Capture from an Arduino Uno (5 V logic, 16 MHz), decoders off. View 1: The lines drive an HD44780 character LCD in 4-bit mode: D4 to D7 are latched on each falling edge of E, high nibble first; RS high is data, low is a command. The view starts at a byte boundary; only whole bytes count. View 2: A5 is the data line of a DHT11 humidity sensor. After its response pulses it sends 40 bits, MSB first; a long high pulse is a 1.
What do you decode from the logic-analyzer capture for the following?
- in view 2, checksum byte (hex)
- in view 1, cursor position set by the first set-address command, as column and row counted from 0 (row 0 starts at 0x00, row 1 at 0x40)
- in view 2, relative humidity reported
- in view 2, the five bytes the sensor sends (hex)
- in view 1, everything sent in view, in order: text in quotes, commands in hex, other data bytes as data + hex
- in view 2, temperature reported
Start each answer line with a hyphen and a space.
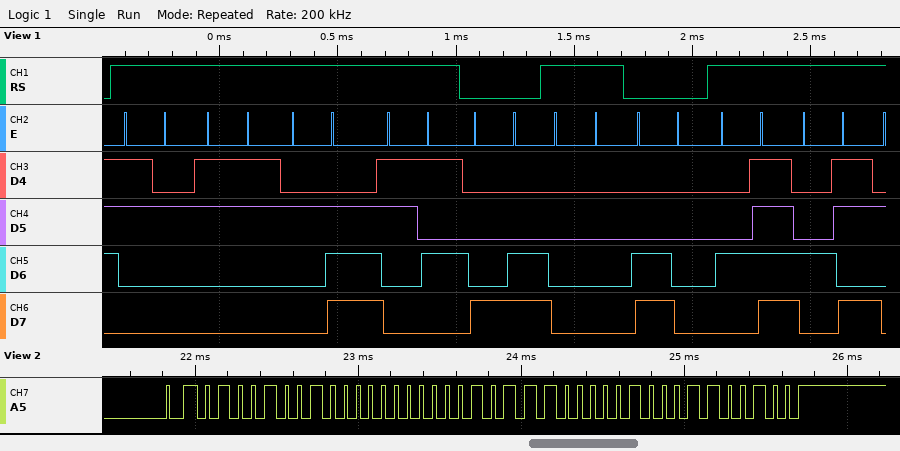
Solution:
- 0x64
- column 12, row 0
- 73 %
- 49 00 17 04 64
- "23.5" 0x8C data 00 0xC0 "OK"
- 23.4 °C
